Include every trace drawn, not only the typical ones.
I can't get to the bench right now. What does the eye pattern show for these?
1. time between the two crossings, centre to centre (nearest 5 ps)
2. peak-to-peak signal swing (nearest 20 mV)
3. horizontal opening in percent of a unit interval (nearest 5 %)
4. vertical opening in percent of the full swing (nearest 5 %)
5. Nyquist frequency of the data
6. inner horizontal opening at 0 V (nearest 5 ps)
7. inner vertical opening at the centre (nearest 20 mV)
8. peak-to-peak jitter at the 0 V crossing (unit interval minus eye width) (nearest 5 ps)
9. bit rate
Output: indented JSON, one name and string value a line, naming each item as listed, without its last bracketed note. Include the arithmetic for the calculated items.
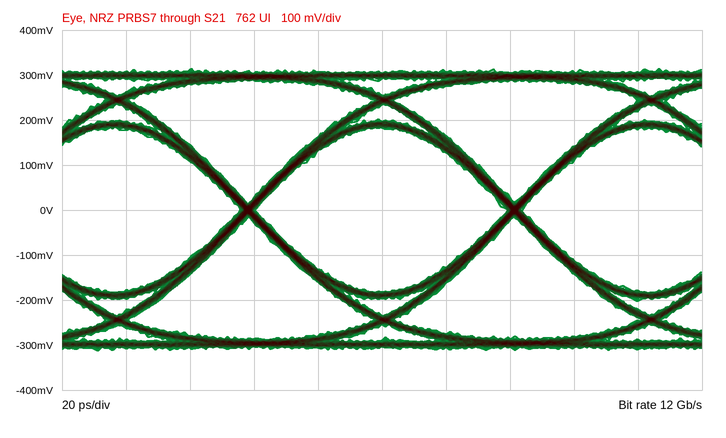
{
  "time between the two crossings, centre to centre": "85 ps",
  "peak-to-peak signal swing": "620 mV",
  "horizontal opening in percent of a unit interval": "80 ps / 85 ps ≈ 94.1 %, so 95 % to the nearest 5 %",
  "vertical opening in percent of the full swing": "360 mV / 620 mV ≈ 58.1 %, so 60 % to the nearest 5 %",
  "Nyquist frequency of the data": "6 GHz",
  "inner horizontal opening at 0 V": "80 ps",
  "inner vertical opening at the centre": "360 mV",
  "peak-to-peak jitter at the 0 V crossing (unit interval minus eye width)": "5 ps",
  "bit rate": "12 Gb/s"
}
